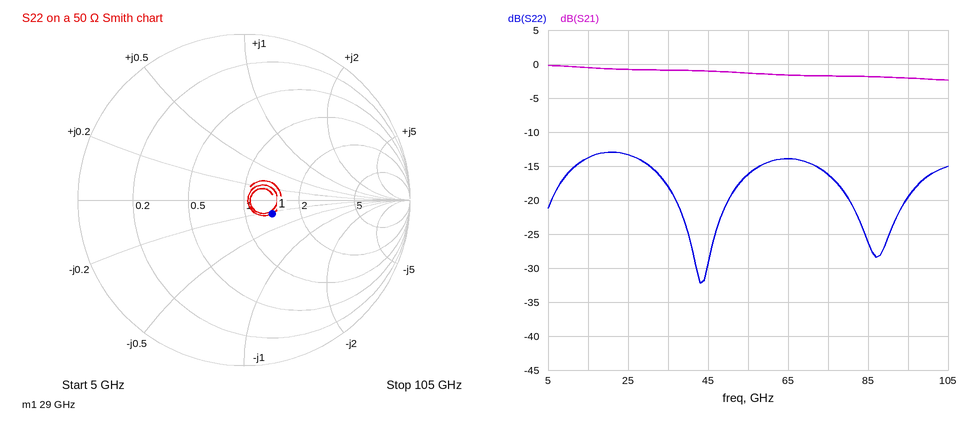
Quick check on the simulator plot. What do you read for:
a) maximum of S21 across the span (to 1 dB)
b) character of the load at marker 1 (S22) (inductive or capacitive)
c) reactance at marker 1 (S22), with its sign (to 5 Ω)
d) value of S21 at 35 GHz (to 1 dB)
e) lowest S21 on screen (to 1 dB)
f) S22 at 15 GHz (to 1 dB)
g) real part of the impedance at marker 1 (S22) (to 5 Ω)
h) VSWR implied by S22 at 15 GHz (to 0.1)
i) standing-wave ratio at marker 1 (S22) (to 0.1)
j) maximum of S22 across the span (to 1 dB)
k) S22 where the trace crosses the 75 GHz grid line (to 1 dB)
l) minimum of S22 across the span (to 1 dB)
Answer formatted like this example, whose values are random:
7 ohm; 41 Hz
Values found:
0 dB; capacitive; -10 Ω; -1 dB; -2 dB; -14 dB; 70 Ω; 1.5; 1.5; -13 dB; -16 dB; -32 dB
